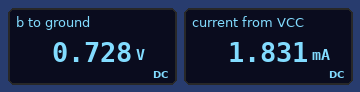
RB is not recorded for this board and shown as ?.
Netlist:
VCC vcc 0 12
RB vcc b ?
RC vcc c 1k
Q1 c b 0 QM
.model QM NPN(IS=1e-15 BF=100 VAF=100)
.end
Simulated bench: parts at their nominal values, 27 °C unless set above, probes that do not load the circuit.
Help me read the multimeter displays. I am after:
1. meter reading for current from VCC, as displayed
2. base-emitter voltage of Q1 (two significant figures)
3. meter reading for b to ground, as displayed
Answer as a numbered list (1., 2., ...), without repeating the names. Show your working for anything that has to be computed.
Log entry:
1. 1.831 mA
2. 728 mV = 730 mV
3. 0.728 V
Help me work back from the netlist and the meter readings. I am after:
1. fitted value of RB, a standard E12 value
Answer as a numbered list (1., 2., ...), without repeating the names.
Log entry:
1. 680 kΩ
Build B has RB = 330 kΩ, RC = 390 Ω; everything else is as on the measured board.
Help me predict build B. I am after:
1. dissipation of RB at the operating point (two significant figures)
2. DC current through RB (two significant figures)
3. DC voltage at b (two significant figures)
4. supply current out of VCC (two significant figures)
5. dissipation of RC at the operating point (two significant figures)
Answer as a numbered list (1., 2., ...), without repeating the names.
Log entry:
1. 380 µW
2. 34 µA
3. 750 mV
4. 3.8 mA
5. 5.5 mW
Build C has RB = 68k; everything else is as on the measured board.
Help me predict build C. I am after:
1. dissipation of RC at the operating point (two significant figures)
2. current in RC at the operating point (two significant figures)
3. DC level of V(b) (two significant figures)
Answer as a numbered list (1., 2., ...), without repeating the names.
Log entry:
1. 140 mW
2. 12 mA
3. 780 mV
